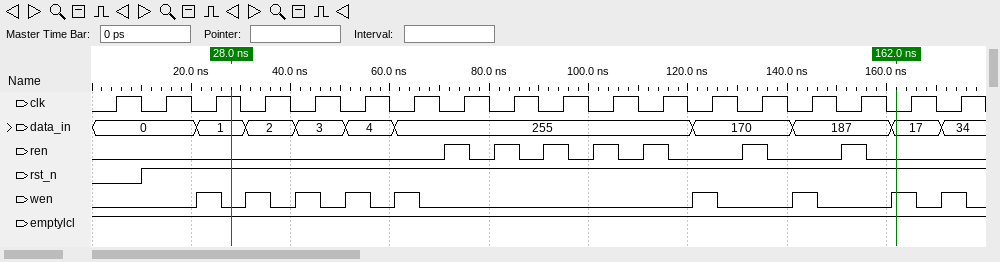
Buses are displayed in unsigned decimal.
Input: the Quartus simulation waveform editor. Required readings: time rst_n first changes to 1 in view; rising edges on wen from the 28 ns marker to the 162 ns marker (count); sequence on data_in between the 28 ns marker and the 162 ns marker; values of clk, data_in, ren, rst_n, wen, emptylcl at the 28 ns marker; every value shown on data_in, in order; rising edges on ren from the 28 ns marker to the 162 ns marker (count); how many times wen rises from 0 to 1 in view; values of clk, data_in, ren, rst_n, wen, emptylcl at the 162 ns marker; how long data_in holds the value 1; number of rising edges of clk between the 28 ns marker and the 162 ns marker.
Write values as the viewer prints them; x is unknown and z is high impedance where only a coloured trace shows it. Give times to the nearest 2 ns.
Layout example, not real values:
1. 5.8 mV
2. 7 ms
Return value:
1. 10 ns
2. 7
3. 1, 2, 3, 4, 255, 170, 187, 17
4. clk=1, data_in=1, ren=0, rst_n=1, wen=0, emptylcl=1
5. 0, 1, 2, 3, 4, 255, 170, 187, 17, 34
6. 7
7. 9
8. clk=0, data_in=17, ren=0, rst_n=1, wen=1, emptylcl=1
9. 10 ns
10. 13
